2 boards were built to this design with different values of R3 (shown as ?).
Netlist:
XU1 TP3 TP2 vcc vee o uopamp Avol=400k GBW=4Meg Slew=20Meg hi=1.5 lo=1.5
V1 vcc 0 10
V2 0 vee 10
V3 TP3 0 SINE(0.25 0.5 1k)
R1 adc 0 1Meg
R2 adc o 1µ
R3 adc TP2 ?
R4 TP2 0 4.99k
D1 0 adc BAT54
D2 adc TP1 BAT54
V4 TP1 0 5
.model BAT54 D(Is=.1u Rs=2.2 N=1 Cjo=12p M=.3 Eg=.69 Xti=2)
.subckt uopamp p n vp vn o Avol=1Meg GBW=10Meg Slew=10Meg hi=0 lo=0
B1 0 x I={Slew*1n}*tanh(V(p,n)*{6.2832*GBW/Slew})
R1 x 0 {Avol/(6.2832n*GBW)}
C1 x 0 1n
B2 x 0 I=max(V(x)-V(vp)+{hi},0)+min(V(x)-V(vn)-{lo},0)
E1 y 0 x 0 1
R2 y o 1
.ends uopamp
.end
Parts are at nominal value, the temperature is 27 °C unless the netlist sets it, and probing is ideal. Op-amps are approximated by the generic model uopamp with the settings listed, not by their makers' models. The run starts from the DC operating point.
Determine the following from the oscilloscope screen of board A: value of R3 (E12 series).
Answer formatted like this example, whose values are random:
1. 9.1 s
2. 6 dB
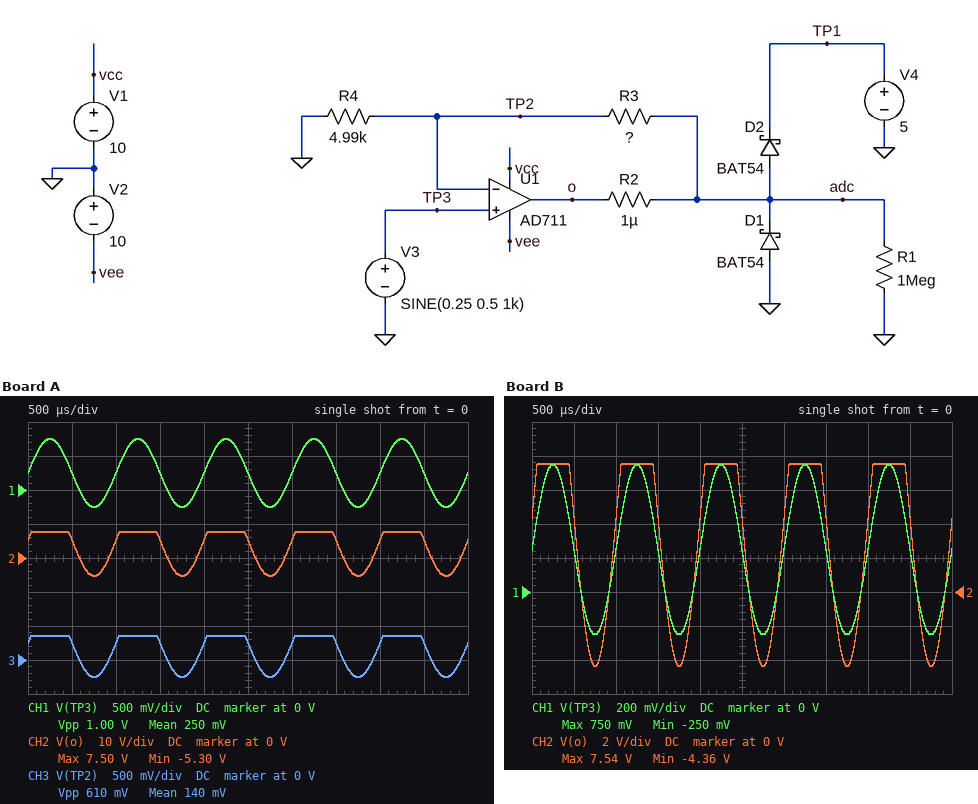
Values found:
1. 100 kΩ
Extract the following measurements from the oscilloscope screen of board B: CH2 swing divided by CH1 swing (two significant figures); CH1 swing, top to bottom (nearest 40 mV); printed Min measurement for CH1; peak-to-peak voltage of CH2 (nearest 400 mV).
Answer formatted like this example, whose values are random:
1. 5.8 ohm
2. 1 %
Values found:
1. 12
2. 1.00 V
3. -250 mV
4. 12.0 V
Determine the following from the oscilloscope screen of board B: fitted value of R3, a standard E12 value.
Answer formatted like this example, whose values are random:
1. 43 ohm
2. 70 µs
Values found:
1. 82 kΩ
